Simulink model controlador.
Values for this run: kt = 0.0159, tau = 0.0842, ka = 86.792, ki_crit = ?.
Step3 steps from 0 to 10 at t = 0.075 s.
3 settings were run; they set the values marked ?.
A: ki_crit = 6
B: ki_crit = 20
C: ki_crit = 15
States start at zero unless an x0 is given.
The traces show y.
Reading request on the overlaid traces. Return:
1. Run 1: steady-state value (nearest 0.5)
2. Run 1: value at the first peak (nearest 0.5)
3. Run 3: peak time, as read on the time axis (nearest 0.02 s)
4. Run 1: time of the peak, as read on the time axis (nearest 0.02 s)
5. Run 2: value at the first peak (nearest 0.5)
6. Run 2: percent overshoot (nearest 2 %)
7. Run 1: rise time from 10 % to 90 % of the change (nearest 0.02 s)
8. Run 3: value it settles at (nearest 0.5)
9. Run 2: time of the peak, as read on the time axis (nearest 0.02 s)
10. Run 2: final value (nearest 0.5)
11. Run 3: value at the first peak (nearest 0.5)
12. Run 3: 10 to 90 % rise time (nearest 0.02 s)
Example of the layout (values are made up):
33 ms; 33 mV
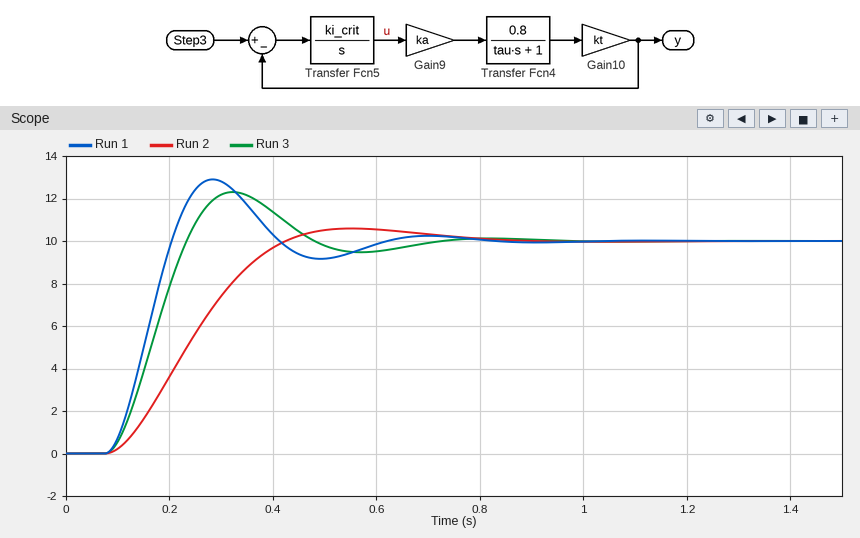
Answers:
10.0; 13.0; 0.32 s; 0.28 s; 10.5; 6 %; 0.08 s; 10.0; 0.56 s; 10.0; 12.5; 0.10 s
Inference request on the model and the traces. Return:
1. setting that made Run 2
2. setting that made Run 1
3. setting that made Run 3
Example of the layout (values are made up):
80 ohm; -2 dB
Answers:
A; B; C
